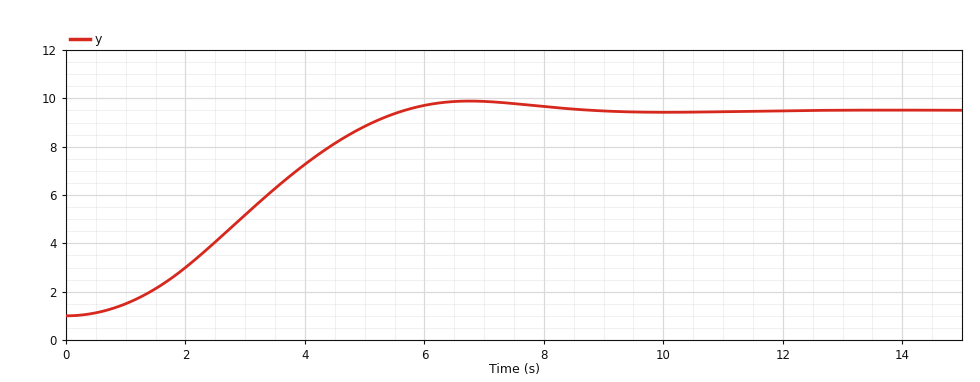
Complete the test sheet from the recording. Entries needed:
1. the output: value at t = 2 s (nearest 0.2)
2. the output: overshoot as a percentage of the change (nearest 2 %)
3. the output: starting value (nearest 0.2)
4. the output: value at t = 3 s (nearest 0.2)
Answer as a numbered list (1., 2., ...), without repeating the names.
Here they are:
1. 3.0
2. 4 %
3. 1.0
4. 5.2
